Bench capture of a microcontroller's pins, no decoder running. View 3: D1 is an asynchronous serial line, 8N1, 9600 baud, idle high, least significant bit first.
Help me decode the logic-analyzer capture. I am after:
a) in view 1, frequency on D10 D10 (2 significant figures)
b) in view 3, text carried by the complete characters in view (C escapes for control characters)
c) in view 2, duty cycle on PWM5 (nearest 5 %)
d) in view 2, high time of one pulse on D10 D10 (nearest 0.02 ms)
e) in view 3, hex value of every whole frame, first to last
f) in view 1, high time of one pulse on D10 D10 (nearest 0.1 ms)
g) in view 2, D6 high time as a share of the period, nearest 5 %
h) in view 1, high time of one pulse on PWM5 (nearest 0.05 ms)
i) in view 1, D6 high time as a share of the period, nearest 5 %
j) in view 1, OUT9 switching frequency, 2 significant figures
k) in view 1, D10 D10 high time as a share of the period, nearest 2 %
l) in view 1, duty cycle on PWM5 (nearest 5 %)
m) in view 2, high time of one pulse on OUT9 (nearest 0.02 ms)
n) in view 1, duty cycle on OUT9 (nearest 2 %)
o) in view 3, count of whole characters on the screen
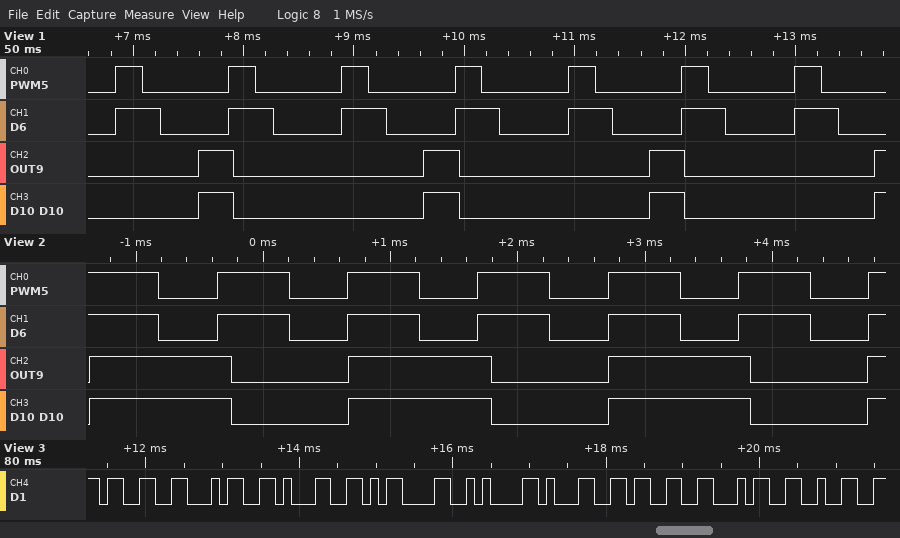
490 Hz
"341\r\n1342"
55 %
1.12 ms
33 34 31 0D 0A 31 33 34 32
0.3 ms
55 %
0.25 ms
40 %
490 Hz
16 %
25 %
1.12 ms
16 %
9
